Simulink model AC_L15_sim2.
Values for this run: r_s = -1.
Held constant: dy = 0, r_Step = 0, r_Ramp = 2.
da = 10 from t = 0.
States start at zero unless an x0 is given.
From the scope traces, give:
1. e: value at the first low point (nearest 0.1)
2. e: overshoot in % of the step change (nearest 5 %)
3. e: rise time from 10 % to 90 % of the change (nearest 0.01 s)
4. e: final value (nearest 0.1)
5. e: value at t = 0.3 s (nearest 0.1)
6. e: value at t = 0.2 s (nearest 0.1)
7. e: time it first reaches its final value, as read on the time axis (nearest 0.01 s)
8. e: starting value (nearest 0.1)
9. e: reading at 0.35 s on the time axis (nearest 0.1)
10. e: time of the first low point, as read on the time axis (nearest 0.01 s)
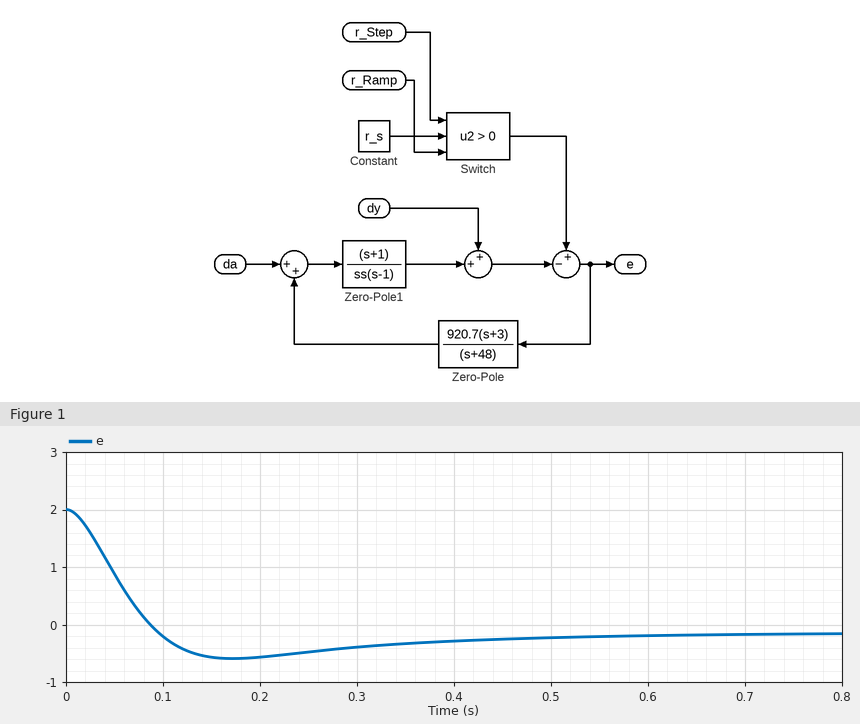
-0.6
20 %
0.07 s
-0.2
-0.4
-0.6
0.10 s
2.0
-0.3
0.17 s
